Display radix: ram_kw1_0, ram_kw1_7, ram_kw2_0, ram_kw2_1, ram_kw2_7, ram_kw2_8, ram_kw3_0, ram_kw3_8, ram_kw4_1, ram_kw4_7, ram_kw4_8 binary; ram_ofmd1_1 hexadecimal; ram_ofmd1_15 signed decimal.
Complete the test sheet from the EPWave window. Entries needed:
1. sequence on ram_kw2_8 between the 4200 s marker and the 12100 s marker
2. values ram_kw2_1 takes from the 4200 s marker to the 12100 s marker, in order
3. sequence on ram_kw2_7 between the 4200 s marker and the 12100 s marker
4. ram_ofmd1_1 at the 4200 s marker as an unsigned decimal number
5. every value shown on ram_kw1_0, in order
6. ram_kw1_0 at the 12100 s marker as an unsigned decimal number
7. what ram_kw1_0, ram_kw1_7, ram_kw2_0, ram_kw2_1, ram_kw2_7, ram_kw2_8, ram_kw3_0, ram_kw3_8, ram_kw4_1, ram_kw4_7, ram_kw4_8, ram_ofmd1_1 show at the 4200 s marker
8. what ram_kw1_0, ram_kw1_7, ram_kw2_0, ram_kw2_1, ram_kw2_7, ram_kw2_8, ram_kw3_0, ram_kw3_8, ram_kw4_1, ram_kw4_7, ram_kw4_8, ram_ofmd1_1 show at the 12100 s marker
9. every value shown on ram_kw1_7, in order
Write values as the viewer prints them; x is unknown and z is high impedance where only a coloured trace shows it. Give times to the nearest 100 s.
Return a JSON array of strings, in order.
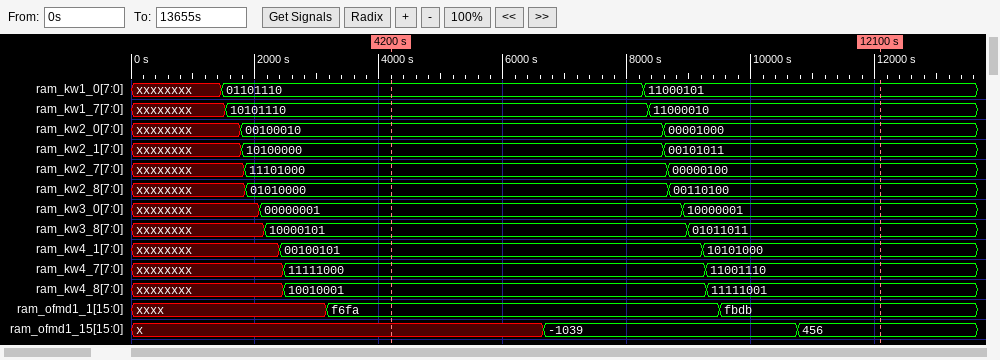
["01010000, 00110100", "10100000, 00101011", "11101000, 00000100", "63226", "xxxxxxxx, 01101110, 11000101", "197", "ram_kw1_0=01101110, ram_kw1_7=10101110, ram_kw2_0=00100010, ram_kw2_1=10100000, ram_kw2_7=11101000, ram_kw2_8=01010000, ram_kw3_0=00000001, ram_kw3_8=10000101, ram_kw4_1=00100101, ram_kw4_7=11111000, ram_kw4_8=10010001, ram_ofmd1_1=f6fa", "ram_kw1_0=11000101, ram_kw1_7=11000010, ram_kw2_0=00001000, ram_kw2_1=00101011, ram_kw2_7=00000100, ram_kw2_8=00110100, ram_kw3_0=10000001, ram_kw3_8=01011011, ram_kw4_1=10101000, ram_kw4_7=11001110, ram_kw4_8=11111001, ram_ofmd1_1=fbdb", "xxxxxxxx, 10101110, 11000010"]
